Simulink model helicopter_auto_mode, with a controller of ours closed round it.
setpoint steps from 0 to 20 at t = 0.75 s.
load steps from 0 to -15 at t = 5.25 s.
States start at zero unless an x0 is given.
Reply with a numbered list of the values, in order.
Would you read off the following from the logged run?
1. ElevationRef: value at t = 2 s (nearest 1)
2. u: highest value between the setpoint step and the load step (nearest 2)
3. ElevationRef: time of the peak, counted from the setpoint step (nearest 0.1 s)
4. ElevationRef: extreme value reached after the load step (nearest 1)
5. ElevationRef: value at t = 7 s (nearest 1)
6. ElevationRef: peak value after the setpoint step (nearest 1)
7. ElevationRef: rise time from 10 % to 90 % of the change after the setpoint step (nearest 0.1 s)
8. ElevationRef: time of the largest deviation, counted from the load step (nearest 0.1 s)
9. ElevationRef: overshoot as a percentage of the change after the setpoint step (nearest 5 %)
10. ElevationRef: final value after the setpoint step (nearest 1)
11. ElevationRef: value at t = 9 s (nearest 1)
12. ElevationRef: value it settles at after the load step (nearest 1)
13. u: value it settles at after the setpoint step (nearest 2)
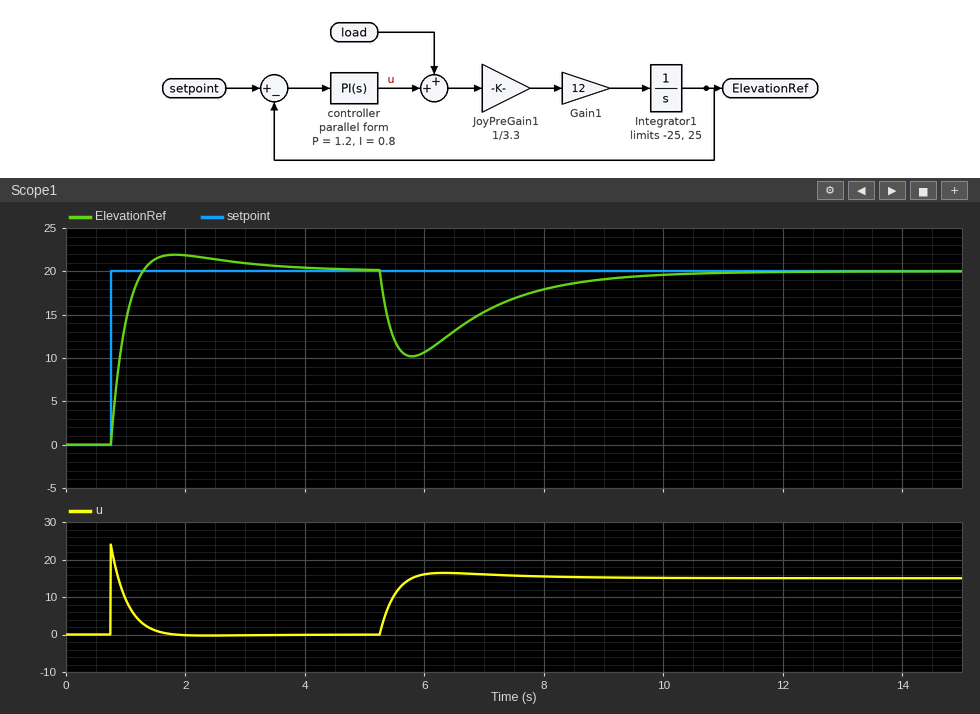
1. 22
2. 24
3. 1.1 s
4. 10
5. 15
6. 22
7. 0.4 s
8. 0.5 s
9. 10 %
10. 20
11. 19
12. 20
13. 0
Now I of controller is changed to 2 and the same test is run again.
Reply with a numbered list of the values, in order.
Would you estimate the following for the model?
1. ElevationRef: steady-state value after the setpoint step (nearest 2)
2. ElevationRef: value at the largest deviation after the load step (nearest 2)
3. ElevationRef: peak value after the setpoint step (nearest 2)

1. 20
2. 12
3. 24
